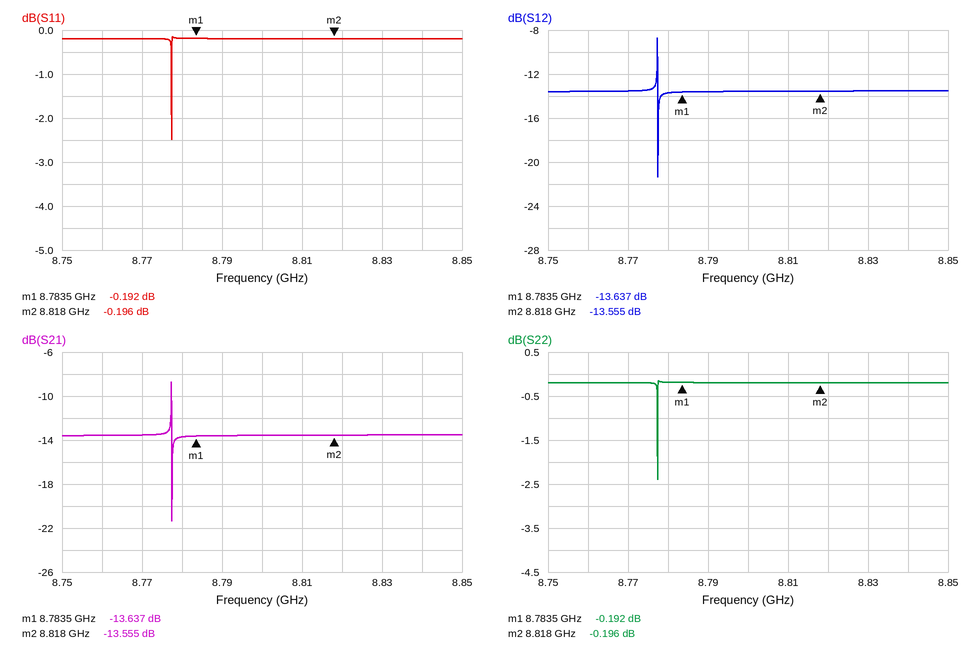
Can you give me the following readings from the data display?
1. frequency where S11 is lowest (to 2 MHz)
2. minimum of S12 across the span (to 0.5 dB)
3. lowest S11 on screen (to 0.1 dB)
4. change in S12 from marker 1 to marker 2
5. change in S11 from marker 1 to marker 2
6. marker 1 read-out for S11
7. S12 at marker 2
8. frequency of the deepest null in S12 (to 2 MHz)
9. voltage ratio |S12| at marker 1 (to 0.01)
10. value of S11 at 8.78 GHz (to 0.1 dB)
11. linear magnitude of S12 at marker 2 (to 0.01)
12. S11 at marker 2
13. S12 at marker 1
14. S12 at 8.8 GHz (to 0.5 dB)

8.778 GHz
-21.5 dB
-2.5 dB
0.082 dB
-0.004 dB
-0.192 dB
-13.555 dB
8.778 GHz
0.21
-0.2 dB
0.21
-0.196 dB
-13.637 dB
-13.5 dB
